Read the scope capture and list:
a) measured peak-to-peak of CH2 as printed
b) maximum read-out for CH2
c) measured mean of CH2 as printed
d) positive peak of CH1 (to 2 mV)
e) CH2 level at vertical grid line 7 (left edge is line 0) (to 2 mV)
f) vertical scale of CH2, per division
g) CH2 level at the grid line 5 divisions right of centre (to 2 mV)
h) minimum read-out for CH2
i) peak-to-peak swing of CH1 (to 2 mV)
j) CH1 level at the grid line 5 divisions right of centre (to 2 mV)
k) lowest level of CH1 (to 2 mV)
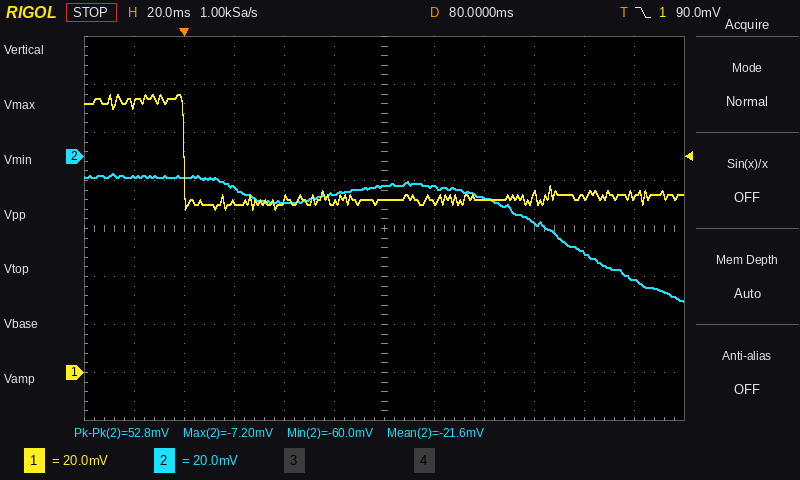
52.8 mV
-7.20 mV
-21.6 mV
116 mV
-12 mV
20 mV
-52 mV
-60.0 mV
48 mV
74 mV
68 mV
